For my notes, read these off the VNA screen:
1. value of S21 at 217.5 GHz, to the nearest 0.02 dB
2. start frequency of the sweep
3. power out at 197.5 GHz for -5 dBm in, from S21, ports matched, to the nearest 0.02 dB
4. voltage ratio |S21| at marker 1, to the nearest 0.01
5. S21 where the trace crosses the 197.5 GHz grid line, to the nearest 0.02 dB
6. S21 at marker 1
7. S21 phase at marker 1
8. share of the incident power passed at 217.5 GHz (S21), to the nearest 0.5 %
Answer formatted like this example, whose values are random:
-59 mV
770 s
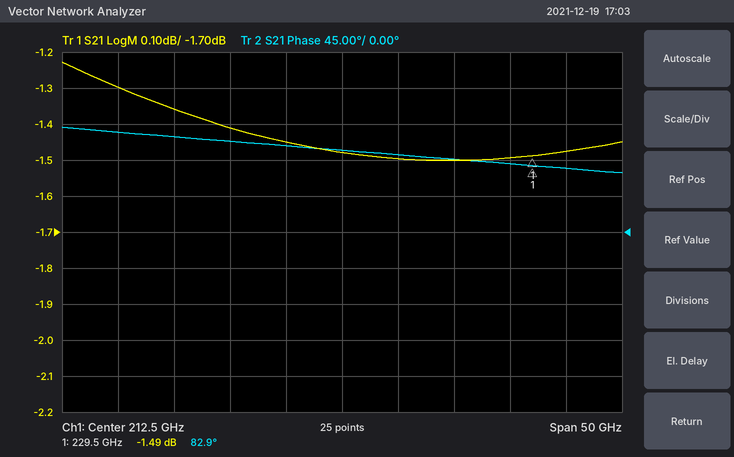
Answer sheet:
-1.50 dB
187.5 GHz
-6.36 dBm
0.84
-1.36 dB
-1.49 dB
82.9°
71.0 %
